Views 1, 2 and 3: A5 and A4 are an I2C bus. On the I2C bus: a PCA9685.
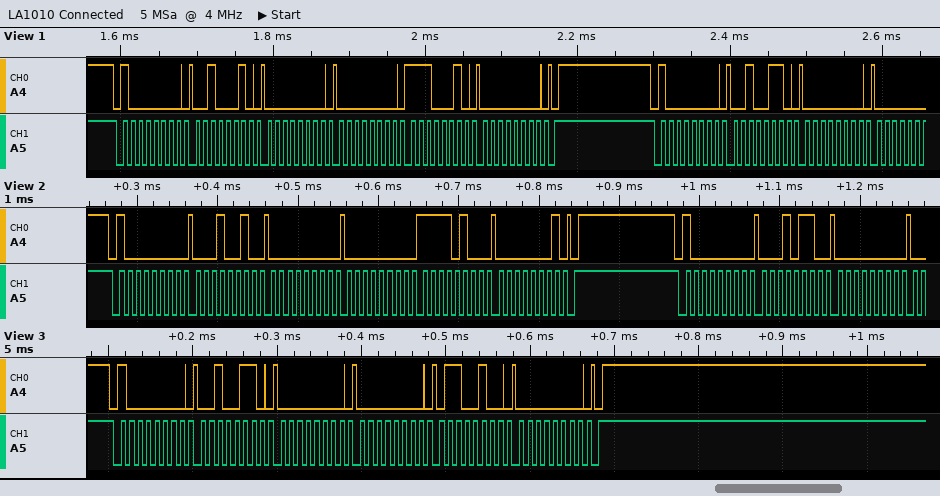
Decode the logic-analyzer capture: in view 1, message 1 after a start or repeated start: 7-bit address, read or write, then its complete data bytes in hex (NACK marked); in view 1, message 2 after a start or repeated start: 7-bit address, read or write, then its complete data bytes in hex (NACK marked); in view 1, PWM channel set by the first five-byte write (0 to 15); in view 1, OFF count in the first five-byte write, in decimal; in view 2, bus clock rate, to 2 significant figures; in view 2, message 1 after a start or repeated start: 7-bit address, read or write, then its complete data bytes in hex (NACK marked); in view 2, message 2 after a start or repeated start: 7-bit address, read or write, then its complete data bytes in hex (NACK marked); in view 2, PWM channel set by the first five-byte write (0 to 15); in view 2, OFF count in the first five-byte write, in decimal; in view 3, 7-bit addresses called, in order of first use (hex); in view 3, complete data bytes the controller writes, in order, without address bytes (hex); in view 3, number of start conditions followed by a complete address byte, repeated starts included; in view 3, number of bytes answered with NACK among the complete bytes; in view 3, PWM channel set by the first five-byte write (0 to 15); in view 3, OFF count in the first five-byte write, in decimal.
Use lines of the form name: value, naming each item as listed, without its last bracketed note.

in view 1, message 1 after a start or repeated start: 7-bit address, read or write, then its complete data bytes in hex: 0x40 write: 22 00 00 E2 00
in view 1, message 2 after a start or repeated start: 7-bit address, read or write, then its complete data bytes in hex: 0x40 write: 26 00
in view 1, PWM channel set by the first five-byte write: 7
in view 1, OFF count in the first five-byte write, in decimal: 226
in view 2, bus clock rate, to 2 significant figures: 100 kHz
in view 2, message 1 after a start or repeated start: 7-bit address, read or write, then its complete data bytes in hex: 0x40 write: 12 00 00 F4 01
in view 2, message 2 after a start or repeated start: 7-bit address, read or write, then its complete data bytes in hex: 0x40 write: 16 00
in view 2, PWM channel set by the first five-byte write: 3
in view 2, OFF count in the first five-byte write, in decimal: 500
in view 3, 7-bit addresses called, in order of first use: 0x40
in view 3, complete data bytes the controller writes, in order, without address bytes: 26 00 00 64 00
in view 3, number of start conditions followed by a complete address byte, repeated starts included: 1
in view 3, number of bytes answered with NACK among the complete bytes: 0
in view 3, PWM channel set by the first five-byte write: 8
in view 3, OFF count in the first five-byte write, in decimal: 100
